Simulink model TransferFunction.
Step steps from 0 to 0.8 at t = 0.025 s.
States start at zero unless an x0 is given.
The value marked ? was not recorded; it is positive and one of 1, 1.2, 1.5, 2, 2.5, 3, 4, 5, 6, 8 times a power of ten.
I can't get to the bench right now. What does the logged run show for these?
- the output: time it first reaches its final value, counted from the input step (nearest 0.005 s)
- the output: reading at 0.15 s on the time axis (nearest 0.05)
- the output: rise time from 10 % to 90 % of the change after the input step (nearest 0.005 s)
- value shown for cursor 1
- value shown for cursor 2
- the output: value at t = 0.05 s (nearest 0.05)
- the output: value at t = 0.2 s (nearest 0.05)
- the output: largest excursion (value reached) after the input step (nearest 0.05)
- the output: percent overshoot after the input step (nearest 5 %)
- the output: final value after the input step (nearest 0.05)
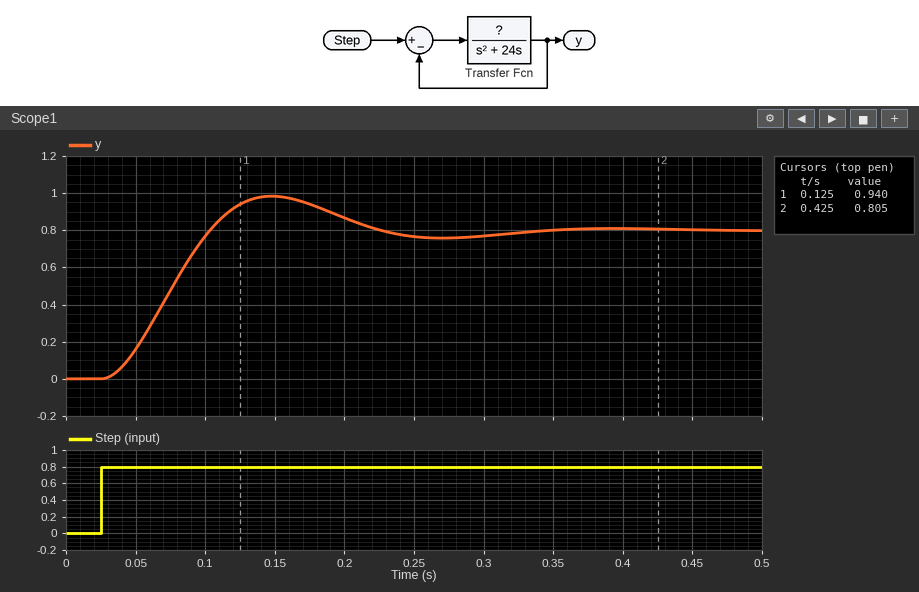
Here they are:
0.080 s
1.00
0.055 s
0.940
0.805
0.15
0.85
1.00
25 %
0.80
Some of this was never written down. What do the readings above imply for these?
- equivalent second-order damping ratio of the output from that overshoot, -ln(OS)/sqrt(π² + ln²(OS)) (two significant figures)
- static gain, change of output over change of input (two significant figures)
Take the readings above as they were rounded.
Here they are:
0.40
1.0
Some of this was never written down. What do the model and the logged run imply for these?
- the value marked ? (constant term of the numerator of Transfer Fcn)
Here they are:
800
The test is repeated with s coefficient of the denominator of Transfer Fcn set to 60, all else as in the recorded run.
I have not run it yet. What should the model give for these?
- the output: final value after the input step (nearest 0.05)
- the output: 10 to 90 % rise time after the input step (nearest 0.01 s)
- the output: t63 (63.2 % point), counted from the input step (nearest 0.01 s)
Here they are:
0.80
0.13 s
0.08 s
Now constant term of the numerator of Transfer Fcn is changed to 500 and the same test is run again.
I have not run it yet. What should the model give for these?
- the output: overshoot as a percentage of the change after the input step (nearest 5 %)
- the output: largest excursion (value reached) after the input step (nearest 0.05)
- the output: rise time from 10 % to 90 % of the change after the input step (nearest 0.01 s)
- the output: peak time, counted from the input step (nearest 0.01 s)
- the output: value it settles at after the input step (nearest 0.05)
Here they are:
15 %
0.90
0.08 s
0.17 s
0.80
